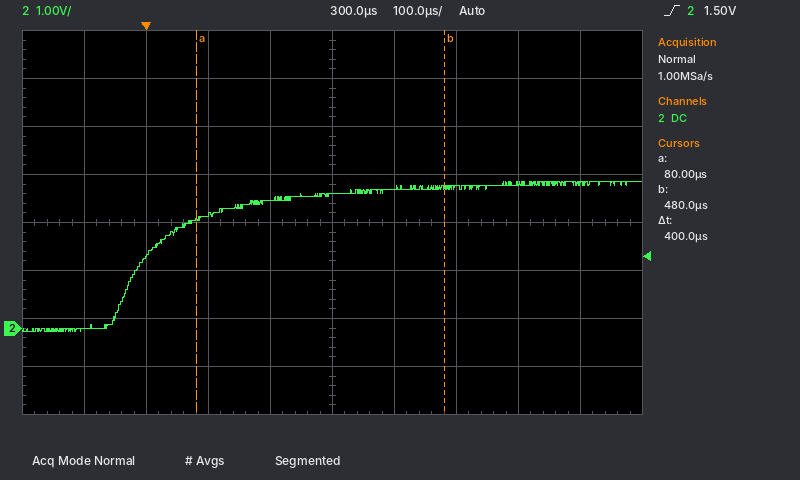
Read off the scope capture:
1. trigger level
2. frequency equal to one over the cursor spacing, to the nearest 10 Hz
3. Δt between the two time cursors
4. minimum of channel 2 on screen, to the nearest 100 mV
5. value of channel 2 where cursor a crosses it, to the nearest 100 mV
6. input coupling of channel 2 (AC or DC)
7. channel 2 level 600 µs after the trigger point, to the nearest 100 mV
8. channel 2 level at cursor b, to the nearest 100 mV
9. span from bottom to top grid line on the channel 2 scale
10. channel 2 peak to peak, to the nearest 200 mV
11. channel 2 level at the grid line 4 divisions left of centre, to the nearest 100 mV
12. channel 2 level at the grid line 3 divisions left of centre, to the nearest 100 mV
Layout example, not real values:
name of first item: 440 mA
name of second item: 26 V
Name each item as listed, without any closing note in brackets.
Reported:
trigger level: 1.50 V
frequency equal to one over the cursor spacing, to the nearest 10 Hz: 2.50 kHz
Δt between the two time cursors: 400 µs
minimum of channel 2 on screen, to the nearest 100 mV: -100 mV
value of channel 2 where cursor a crosses it, to the nearest 100 mV: 2.3 V
input coupling of channel 2: DC
channel 2 level 600 µs after the trigger point, to the nearest 100 mV: 3.0 V
channel 2 level at cursor b, to the nearest 100 mV: 2.9 V
span from bottom to top grid line on the channel 2 scale: 8 V
channel 2 peak to peak, to the nearest 200 mV: 3.2 V
channel 2 level at the grid line 4 divisions left of centre, to the nearest 100 mV: 0.0 V
channel 2 level at the grid line 3 divisions left of centre, to the nearest 100 mV: 1.5 V
